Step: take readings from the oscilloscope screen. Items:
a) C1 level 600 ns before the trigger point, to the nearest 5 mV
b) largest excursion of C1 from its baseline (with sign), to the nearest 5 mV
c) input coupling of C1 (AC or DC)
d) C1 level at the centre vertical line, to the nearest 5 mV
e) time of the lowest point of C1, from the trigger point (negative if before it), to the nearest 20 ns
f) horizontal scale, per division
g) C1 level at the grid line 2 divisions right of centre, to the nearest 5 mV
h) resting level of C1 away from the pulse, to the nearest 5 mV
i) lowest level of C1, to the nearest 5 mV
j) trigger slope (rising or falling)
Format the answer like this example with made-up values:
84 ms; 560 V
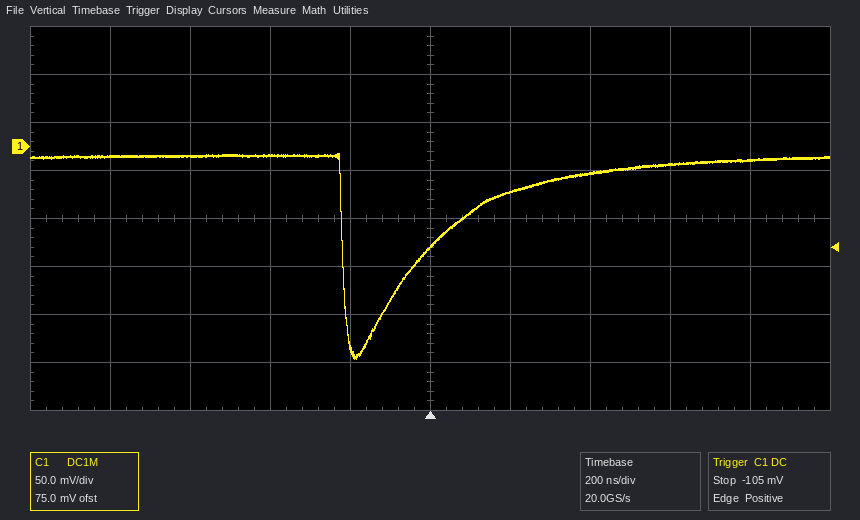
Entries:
-10 mV; -210 mV; DC; -105 mV; -180 ns; 200 ns; -30 mV; -10 mV; -220 mV; rising
